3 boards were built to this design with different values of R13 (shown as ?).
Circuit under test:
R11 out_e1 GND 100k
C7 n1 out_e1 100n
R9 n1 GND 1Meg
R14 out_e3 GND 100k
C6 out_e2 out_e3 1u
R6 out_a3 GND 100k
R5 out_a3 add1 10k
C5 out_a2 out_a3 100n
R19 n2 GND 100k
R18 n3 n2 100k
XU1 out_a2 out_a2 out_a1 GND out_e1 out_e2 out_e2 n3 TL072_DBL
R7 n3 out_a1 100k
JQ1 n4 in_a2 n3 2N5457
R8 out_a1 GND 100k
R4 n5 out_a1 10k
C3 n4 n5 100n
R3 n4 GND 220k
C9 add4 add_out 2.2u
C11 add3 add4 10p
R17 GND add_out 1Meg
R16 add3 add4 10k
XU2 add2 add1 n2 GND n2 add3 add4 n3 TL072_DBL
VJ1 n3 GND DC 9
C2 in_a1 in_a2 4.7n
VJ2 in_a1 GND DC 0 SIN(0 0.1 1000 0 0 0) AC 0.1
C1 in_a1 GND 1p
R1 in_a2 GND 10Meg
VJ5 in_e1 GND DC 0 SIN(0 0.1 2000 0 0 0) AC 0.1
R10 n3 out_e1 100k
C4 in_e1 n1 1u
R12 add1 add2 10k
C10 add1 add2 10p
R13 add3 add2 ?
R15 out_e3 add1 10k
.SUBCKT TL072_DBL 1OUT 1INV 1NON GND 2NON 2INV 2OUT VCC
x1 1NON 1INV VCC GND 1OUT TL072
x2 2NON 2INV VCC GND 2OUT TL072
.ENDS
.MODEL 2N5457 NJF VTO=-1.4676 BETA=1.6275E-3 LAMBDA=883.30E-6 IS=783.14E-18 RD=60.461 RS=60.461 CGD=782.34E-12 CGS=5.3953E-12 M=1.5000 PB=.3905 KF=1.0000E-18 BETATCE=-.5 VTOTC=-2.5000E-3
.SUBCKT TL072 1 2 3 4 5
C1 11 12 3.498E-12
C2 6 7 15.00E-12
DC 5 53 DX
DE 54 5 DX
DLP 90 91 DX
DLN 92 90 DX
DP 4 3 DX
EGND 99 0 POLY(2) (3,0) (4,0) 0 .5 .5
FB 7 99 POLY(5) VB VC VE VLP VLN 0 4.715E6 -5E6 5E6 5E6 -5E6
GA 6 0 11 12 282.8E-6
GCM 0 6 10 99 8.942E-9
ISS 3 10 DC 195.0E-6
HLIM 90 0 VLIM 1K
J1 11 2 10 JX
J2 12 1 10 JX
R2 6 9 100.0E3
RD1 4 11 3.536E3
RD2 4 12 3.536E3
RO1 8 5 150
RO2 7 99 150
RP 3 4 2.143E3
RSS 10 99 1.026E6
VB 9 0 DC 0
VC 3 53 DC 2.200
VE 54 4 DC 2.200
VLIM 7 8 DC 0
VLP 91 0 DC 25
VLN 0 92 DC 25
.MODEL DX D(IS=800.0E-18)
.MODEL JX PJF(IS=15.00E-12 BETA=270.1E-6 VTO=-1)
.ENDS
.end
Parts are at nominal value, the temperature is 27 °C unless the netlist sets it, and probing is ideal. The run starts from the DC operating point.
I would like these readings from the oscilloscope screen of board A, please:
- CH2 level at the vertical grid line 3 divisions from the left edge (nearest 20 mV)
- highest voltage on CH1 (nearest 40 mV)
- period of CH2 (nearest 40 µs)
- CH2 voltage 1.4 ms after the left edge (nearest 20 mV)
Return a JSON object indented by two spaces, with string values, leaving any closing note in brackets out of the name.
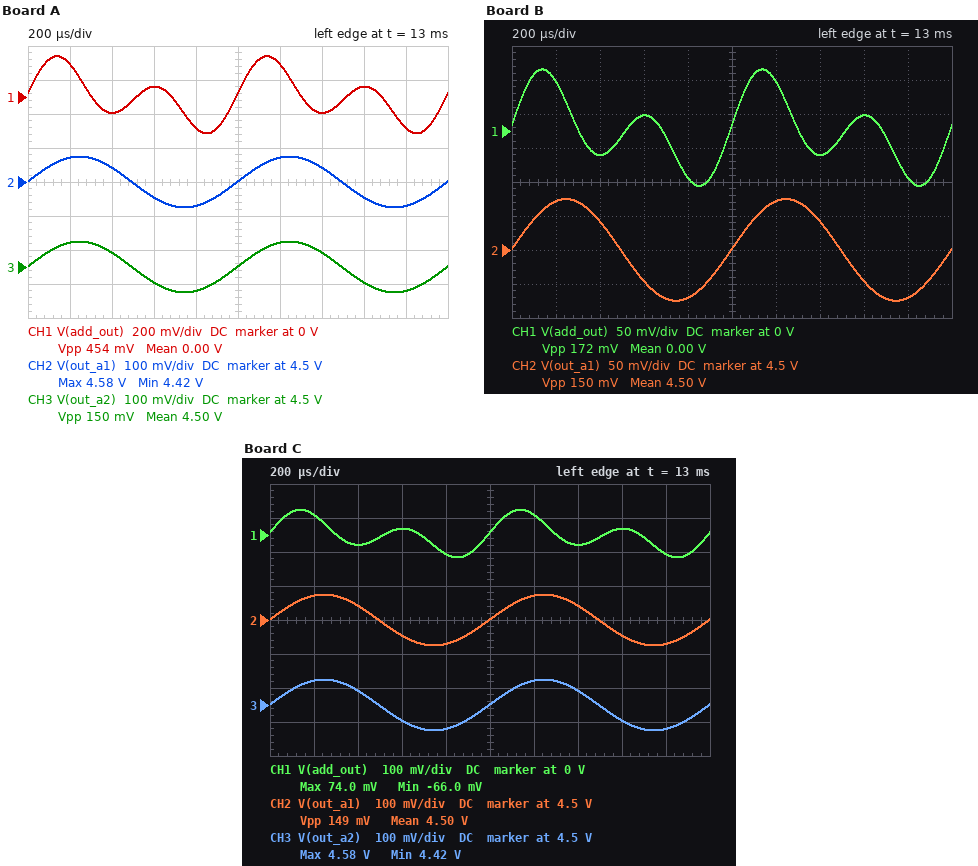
{
  "CH2 level at the vertical grid line 3 divisions from the left edge": "4.46 V",
  "highest voltage on CH1": "240 mV",
  "period of CH2": "1.00 ms",
  "CH2 voltage 1.4 ms after the left edge": "4.54 V"
}
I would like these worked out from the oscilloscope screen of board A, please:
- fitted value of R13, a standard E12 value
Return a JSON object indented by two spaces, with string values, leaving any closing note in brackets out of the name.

{
  "fitted value of R13, a standard E12 value": "6.8 kΩ"
}
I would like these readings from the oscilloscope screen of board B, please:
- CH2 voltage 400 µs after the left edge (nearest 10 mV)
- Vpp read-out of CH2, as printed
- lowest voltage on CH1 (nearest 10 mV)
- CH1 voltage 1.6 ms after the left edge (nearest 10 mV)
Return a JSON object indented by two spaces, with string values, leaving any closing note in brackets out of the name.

{
  "CH2 voltage 400 µs after the left edge": "4.54 V",
  "Vpp read-out of CH2, as printed": "150 mV",
  "lowest voltage on CH1": "-80 mV",
  "CH1 voltage 1.6 ms after the left edge": "20 mV"
}
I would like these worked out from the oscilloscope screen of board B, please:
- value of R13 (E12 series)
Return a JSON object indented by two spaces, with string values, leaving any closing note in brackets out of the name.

{
  "value of R13": "18 kΩ"
}
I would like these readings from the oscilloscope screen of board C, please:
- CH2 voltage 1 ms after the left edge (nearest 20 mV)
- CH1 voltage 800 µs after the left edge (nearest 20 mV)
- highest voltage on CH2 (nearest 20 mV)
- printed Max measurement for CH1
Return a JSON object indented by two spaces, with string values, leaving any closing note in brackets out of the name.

{
  "CH2 voltage 1 ms after the left edge": "4.50 V",
  "CH1 voltage 800 µs after the left edge": "-60 mV",
  "highest voltage on CH2": "4.58 V",
  "printed Max measurement for CH1": "74.0 mV"
}
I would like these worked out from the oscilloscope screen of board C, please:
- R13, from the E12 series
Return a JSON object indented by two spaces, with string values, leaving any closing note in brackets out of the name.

{
  "R13, from the E12 series": "22 kΩ"
}
